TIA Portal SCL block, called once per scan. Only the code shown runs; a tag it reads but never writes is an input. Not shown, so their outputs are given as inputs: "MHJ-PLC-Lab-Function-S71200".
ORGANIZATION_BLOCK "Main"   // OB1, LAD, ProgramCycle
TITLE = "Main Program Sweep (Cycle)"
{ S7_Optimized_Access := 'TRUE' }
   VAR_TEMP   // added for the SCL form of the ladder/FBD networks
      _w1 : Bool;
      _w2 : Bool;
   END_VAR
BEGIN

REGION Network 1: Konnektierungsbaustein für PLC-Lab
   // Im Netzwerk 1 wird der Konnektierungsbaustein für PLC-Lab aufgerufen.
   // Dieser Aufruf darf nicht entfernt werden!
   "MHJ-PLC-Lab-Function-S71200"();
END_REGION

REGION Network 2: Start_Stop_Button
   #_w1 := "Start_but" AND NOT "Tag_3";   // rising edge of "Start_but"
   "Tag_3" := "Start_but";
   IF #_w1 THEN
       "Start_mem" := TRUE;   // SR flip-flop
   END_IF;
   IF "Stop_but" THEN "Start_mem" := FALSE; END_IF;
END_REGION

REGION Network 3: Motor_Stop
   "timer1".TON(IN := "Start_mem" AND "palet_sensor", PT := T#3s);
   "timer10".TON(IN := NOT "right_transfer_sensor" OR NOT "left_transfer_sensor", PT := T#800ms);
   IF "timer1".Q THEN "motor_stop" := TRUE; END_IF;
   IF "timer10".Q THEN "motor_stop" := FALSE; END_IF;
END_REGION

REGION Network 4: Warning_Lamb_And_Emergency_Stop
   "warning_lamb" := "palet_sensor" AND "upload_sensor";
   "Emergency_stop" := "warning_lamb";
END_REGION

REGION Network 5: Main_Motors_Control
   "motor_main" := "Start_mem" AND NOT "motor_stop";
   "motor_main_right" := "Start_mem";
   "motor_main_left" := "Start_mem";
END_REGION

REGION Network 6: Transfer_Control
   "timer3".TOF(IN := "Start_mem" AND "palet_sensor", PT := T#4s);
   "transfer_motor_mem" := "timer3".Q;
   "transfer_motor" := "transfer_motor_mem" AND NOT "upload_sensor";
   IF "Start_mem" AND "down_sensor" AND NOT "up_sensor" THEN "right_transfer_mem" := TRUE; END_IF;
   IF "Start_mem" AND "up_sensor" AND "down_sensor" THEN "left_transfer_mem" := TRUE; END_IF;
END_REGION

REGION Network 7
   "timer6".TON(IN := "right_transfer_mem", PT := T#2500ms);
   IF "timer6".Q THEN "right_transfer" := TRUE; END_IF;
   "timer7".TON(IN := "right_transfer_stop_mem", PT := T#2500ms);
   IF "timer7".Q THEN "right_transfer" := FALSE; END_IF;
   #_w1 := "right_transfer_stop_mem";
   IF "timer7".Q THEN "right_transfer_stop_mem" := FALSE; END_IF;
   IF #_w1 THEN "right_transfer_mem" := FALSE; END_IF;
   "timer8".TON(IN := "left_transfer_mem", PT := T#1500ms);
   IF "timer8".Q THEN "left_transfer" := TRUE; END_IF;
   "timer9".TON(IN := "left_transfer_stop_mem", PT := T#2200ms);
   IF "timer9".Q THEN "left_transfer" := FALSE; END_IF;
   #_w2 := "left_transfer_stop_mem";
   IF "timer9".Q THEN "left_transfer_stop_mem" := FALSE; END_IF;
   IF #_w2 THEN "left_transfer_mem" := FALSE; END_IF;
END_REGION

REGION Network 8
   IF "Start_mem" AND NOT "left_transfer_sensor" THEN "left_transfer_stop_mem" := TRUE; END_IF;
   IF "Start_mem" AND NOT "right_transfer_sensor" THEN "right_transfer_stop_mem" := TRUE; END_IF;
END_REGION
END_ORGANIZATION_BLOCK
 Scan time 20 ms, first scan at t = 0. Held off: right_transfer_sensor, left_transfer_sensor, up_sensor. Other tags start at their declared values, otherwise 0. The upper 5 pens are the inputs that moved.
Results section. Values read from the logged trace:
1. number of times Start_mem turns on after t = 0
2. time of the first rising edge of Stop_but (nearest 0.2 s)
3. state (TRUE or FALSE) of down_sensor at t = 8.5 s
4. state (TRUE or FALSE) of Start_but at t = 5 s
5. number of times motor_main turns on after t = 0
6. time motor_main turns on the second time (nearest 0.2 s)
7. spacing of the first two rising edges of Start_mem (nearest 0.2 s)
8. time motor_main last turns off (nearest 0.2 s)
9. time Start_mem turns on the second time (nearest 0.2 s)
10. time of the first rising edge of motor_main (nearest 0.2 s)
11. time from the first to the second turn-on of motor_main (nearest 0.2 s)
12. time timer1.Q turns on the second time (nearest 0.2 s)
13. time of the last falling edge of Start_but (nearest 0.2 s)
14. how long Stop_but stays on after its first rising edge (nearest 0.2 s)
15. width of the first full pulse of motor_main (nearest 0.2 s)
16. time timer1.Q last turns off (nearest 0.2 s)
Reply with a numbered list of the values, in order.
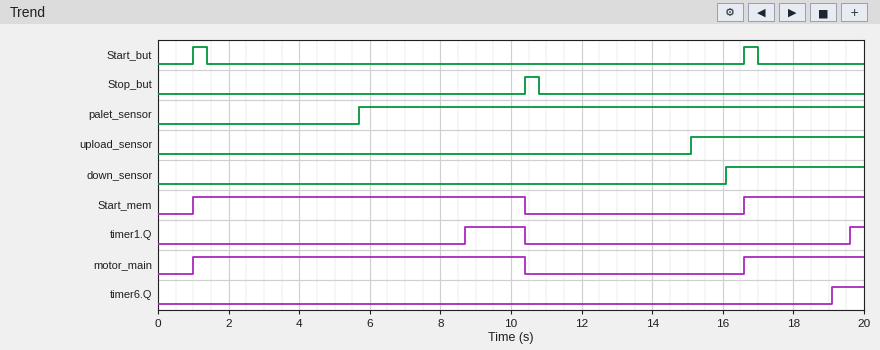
1. 2
2. 10.4 s
3. FALSE
4. FALSE
5. 2
6. 16.6 s
7. 15.6 s
8. 10.4 s
9. 16.6 s
10. 1.0 s
11. 15.6 s
12. 19.6 s
13. 17.0 s
14. 0.4 s
15. 9.4 s
16. 10.4 s
